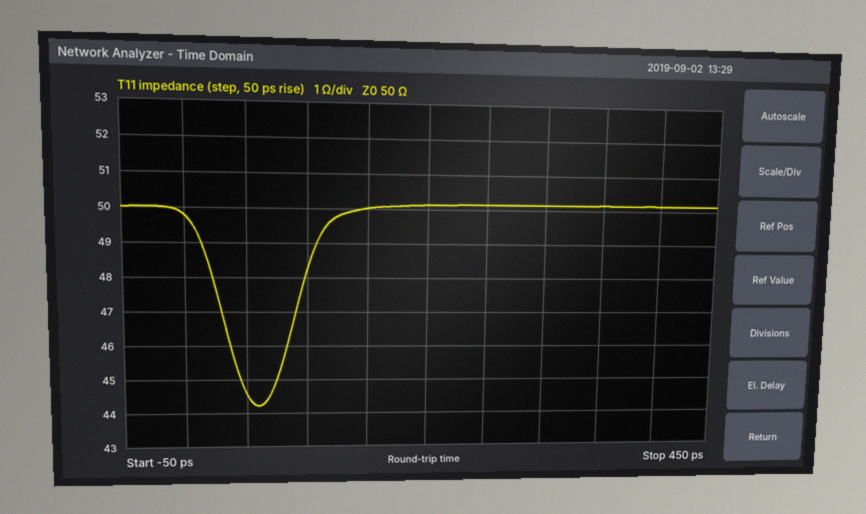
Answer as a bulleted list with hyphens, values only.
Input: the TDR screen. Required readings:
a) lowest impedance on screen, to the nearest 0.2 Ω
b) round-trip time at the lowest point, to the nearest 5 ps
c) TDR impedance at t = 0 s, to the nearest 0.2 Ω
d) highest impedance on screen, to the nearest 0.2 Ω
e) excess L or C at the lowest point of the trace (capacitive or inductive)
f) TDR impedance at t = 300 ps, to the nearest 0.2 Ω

- 44.2 Ω
- 60 ps
- 49.8 Ω
- 50.2 Ω
- capacitive
- 50.2 Ω
